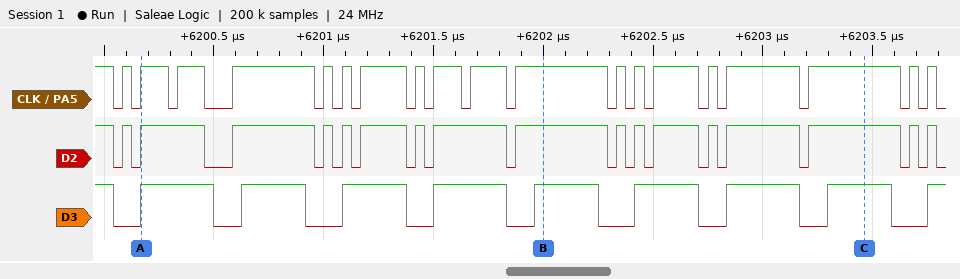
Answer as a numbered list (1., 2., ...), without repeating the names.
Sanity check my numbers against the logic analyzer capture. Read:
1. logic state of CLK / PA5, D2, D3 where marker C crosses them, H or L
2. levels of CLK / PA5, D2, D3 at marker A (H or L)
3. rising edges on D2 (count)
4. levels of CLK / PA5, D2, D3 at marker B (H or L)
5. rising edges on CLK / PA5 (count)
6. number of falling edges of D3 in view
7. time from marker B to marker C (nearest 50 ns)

1. CLK / PA5=H, D2=H, D3=H
2. CLK / PA5=H, D2=H, D3=H
3. 17
4. CLK / PA5=H, D2=H, D3=H
5. 19
6. 9
7. 1450 ns
